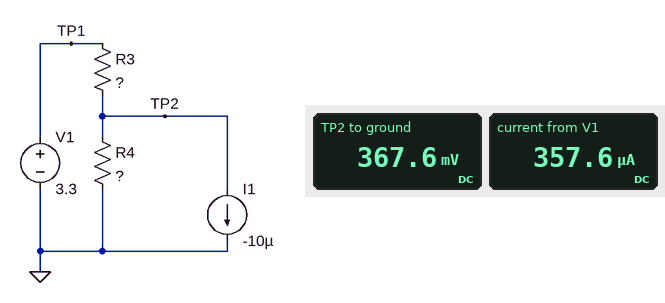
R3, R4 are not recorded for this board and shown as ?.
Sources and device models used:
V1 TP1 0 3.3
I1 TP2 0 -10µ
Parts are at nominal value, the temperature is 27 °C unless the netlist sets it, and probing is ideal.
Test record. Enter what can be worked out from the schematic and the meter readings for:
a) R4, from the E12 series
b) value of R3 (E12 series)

1 kΩ
8.2 kΩ
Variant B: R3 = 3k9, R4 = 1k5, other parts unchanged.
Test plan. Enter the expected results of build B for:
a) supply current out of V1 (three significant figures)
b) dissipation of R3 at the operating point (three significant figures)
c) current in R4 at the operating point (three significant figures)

608 µA
1.44 mW
618 µA
